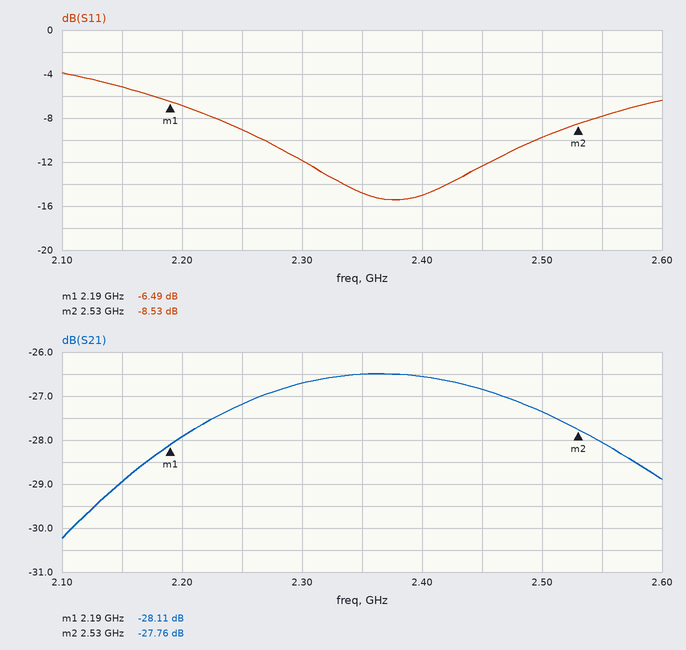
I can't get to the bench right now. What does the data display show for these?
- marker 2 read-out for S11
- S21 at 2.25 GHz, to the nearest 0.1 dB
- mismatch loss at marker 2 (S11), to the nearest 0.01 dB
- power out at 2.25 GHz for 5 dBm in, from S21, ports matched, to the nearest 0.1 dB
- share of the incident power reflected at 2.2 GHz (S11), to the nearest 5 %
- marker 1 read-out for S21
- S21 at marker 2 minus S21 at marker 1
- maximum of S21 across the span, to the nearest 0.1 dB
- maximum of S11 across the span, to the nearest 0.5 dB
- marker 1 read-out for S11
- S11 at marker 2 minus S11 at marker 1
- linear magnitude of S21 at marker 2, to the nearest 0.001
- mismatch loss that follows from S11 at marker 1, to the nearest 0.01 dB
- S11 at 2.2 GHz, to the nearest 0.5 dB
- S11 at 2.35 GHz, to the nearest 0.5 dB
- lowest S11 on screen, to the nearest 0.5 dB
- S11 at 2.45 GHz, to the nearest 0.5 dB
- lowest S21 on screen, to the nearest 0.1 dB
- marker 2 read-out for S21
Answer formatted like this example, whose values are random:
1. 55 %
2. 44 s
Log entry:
1. -8.53 dB
2. -27.2 dB
3. 0.66 dB
4. -22.2 dBm
5. 20 %
6. -28.11 dB
7. 0.35 dB
8. -26.5 dB
9. -4.0 dB
10. -6.49 dB
11. -2.04 dB
12. 0.041
13. 1.10 dB
14. -7.0 dB
15. -15.0 dB
16. -15.5 dB
17. -12.5 dB
18. -30.2 dB
19. -27.76 dB
